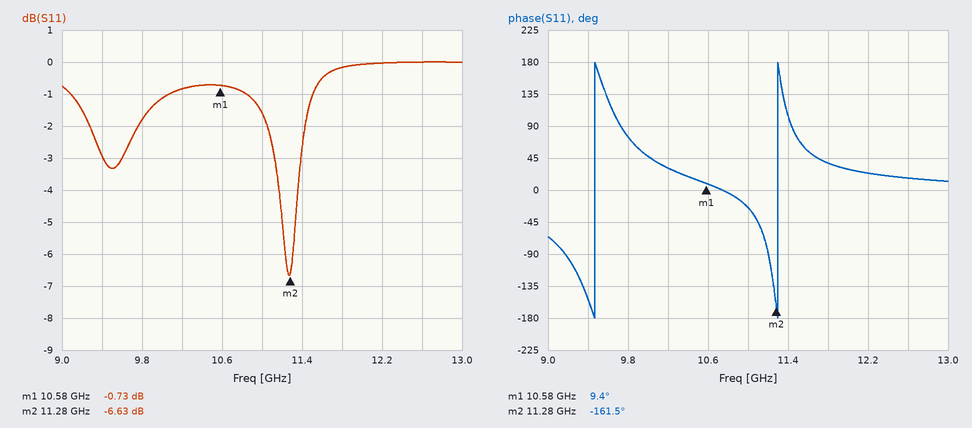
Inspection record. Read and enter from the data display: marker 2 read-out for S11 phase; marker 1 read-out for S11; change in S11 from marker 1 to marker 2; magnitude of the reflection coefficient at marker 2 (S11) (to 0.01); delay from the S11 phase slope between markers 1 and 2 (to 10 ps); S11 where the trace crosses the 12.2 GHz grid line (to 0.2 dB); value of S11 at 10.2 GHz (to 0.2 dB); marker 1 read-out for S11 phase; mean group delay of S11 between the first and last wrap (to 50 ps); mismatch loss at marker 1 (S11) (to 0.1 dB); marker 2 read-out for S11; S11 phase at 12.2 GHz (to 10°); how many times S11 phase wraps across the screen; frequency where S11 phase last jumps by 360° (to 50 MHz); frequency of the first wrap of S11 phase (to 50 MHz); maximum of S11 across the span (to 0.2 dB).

-161.5°
-0.73 dB
-5.90 dB
0.47
680 ps
0.0 dB
-0.8 dB
9.4°
550 ps
8.1 dB
-6.63 dB
20°
2
11.30 GHz
9.45 GHz
0.0 dB
